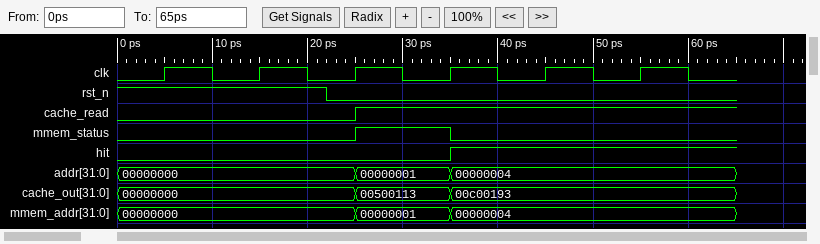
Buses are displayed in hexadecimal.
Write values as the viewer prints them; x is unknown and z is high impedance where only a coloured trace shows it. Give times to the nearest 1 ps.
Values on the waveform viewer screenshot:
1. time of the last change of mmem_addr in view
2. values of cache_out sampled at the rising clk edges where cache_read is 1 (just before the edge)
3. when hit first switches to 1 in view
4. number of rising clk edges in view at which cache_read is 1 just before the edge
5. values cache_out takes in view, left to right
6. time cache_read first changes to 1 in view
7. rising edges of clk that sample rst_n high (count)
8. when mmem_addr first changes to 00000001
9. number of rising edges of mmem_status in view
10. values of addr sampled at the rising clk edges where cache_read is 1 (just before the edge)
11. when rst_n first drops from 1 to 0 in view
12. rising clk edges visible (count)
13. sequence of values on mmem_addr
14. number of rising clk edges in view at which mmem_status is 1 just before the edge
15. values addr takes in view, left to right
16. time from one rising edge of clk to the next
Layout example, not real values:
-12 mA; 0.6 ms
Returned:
35 ps; 00500113, 00c00193, 00c00193; 35 ps; 3; 00000000, 00500113, 00c00193; 25 ps; 2; 25 ps; 1; 00000001, 00000004, 00000004; 22 ps; 6; 00000000, 00000001, 00000004; 1; 00000000, 00000001, 00000004; 10 ps
